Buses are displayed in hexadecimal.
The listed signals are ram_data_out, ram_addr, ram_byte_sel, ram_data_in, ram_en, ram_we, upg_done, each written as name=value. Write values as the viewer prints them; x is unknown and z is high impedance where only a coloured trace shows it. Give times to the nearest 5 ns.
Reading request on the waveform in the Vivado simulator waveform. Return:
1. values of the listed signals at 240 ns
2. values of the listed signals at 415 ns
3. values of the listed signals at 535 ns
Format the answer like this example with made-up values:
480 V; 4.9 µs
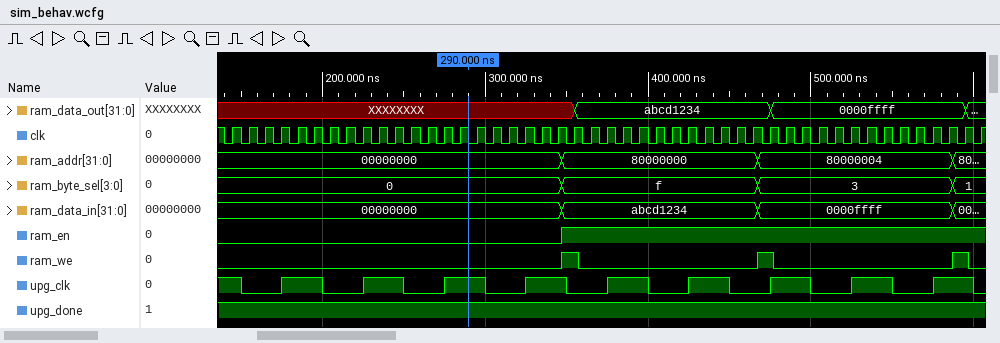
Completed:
ram_data_out=XXXXXXXX, ram_addr=00000000, ram_byte_sel=0, ram_data_in=00000000, ram_en=0, ram_we=0, upg_done=1; ram_data_out=abcd1234, ram_addr=80000000, ram_byte_sel=f, ram_data_in=abcd1234, ram_en=1, ram_we=0, upg_done=1; ram_data_out=0000ffff, ram_addr=80000004, ram_byte_sel=3, ram_data_in=0000ffff, ram_en=1, ram_we=0, upg_done=1
